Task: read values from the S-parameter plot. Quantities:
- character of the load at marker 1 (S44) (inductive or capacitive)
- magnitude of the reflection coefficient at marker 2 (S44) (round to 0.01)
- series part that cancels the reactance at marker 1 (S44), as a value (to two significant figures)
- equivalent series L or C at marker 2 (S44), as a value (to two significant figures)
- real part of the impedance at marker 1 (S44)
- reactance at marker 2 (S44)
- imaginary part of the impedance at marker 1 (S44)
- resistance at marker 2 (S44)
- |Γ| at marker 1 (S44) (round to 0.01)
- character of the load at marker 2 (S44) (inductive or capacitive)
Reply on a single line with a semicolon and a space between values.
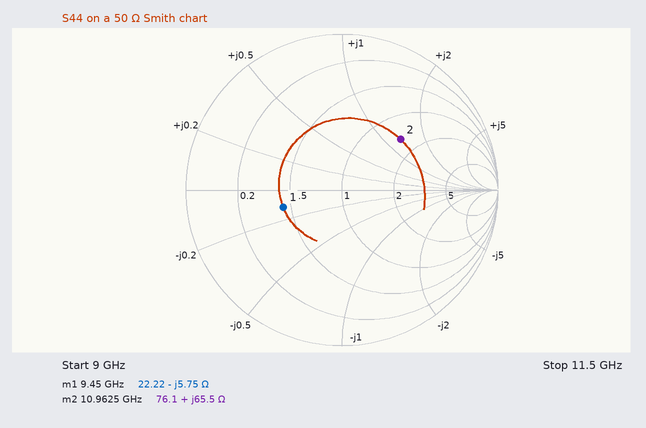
capacitive; 0.50; 97 pH; 950 pH; 22.22 Ω; +65.5 Ω; -5.75 Ω; 76.1 Ω; 0.39; inductive
